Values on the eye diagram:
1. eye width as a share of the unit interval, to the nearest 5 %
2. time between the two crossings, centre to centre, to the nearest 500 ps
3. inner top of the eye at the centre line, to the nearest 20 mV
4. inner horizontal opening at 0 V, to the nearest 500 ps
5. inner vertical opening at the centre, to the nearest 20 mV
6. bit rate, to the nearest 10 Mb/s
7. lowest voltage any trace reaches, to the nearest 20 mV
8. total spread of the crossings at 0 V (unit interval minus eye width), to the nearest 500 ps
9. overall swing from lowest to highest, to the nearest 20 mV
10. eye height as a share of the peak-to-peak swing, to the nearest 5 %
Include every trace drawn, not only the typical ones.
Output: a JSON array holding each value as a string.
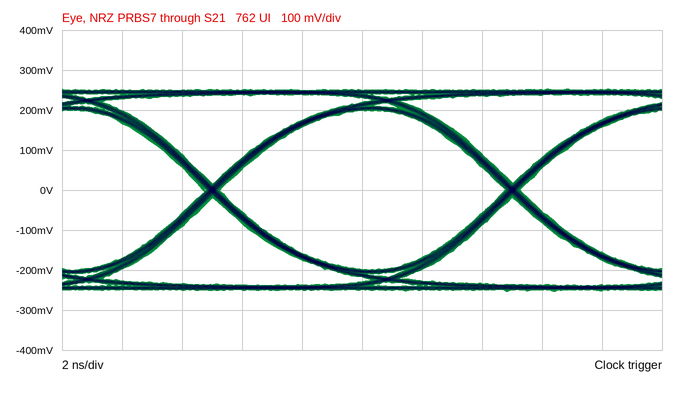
["95 %", "10.0 ns", "200 mV", "9.5 ns", "400 mV", "100 Mb/s", "-260 mV", "500 ps", "500 mV", "80 %"]
